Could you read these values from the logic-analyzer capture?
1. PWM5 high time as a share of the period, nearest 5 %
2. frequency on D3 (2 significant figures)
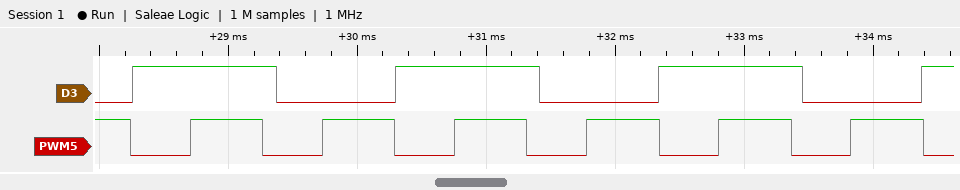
55 %
490 Hz
